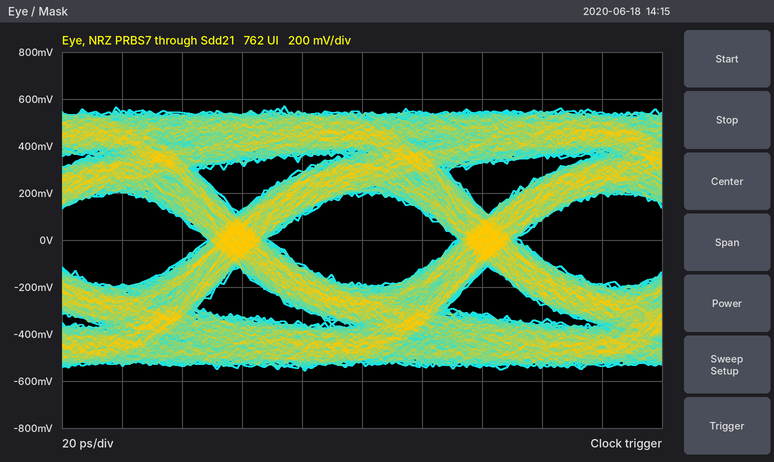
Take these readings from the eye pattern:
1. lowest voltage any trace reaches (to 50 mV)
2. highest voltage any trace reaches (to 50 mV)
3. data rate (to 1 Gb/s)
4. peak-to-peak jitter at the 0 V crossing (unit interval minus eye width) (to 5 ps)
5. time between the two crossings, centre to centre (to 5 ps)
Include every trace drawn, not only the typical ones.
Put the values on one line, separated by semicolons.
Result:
-550 mV; 550 mV; 12 Gb/s; 20 ps; 85 ps
